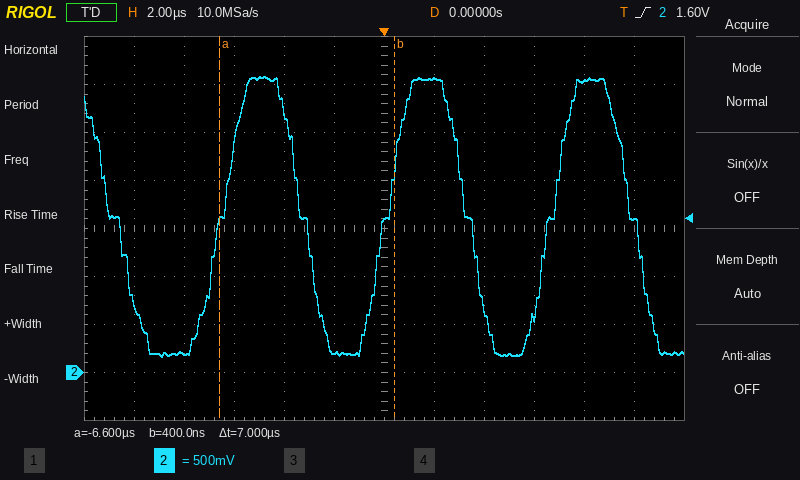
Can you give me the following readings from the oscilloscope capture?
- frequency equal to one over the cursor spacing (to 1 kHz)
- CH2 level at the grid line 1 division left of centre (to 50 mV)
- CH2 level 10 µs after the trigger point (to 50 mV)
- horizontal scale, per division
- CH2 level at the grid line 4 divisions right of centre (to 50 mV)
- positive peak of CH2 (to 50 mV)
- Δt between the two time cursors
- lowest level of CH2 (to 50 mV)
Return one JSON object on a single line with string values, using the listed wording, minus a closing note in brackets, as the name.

{"frequency equal to one over the cursor spacing": "143 kHz", "CH2 level at the grid line 1 division left of centre": "200 mV", "CH2 level 10 µs after the trigger point": "1.60 V", "horizontal scale, per division": "2 µs", "CH2 level at the grid line 4 divisions right of centre": "3.05 V", "positive peak of CH2": "3.10 V", "Δt between the two time cursors": "7 µs", "lowest level of CH2": "150 mV"}
